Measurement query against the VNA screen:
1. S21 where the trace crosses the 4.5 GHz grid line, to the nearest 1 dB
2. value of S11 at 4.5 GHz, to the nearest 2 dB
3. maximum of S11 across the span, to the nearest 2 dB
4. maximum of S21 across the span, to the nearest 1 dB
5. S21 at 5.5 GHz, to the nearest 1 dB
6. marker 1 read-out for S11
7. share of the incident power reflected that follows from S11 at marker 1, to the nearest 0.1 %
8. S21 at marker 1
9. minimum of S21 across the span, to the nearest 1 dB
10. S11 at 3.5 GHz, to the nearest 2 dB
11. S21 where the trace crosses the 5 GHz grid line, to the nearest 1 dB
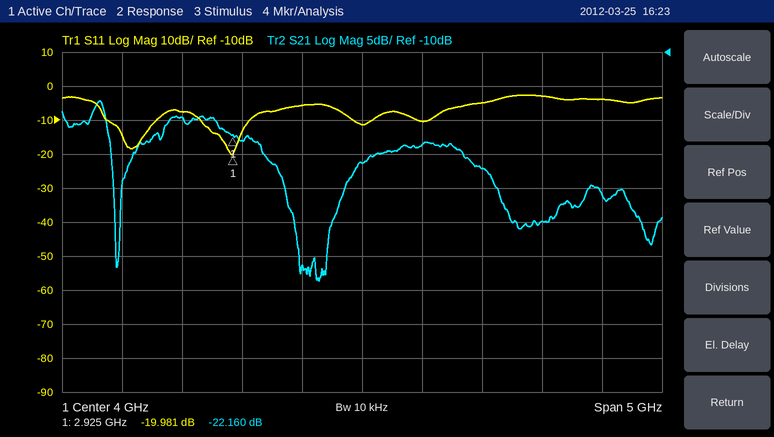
-24 dB
-10 dB
-2 dB
-17 dB
-35 dB
-19.981 dB
1.0 %
-22.160 dB
-44 dB
-6 dB
-27 dB
